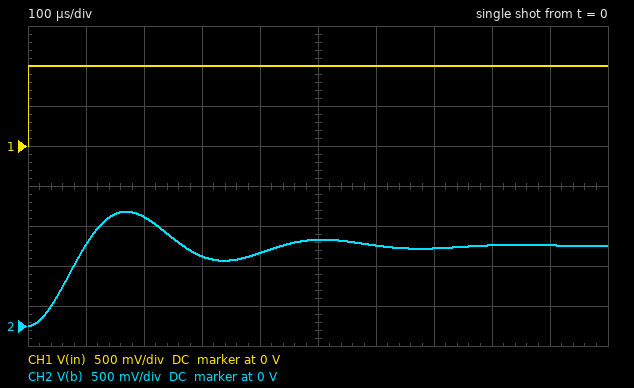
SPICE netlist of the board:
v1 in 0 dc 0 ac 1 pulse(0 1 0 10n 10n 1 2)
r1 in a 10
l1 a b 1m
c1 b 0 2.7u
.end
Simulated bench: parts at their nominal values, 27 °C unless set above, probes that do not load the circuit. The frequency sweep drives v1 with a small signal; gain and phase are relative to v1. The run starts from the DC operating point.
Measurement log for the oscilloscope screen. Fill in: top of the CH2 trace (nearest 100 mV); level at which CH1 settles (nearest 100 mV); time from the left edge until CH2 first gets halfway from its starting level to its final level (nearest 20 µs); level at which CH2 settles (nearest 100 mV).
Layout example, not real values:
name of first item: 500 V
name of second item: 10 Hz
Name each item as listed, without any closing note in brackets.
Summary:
top of the CH2 trace: 1.4 V
level at which CH1 settles: 1.0 V
time from the left edge until CH2 first gets halfway from its starting level to its final level: 60 µs
level at which CH2 settles: 1.0 V
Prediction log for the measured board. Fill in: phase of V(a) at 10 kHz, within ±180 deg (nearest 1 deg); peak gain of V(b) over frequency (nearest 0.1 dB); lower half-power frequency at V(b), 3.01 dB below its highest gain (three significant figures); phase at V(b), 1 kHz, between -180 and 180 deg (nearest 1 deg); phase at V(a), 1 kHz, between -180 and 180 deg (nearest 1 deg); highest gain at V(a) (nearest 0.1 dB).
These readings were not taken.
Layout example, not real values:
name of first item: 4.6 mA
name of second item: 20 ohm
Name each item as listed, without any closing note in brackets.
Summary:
phase of V(a) at 10 kHz, within ±180 deg: 10 deg
peak gain of V(b) over frequency: 6.0 dB
lower half-power frequency at V(b), 3.01 dB below its highest gain: 1.85 kHz
phase at V(b), 1 kHz, between -180 and 180 deg: -11 deg
phase at V(a), 1 kHz, between -180 and 180 deg: -11 deg
highest gain at V(a): 0 dB
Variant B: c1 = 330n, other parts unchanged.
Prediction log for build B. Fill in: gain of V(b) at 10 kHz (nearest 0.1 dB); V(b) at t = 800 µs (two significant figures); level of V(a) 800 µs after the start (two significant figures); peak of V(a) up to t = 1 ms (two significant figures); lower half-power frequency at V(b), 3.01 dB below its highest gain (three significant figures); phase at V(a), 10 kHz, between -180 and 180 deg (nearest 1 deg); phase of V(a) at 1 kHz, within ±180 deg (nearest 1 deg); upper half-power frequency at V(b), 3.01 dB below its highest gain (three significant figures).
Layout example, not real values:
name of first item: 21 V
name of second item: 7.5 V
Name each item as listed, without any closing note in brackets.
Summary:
gain of V(b) at 10 kHz: 8.7 dB
V(b) at t = 800 µs: 980 mV
level of V(a) 800 µs after the start: 1.0 V
peak of V(a) up to t = 1 ms: 1.1 V
lower half-power frequency at V(b), 3.01 dB below its highest gain: 7.85 kHz
phase at V(a), 10 kHz, between -180 and 180 deg: 34 deg
phase of V(a) at 1 kHz, within ±180 deg: -1 deg
upper half-power frequency at V(b), 3.01 dB below its highest gain: 9.45 kHz
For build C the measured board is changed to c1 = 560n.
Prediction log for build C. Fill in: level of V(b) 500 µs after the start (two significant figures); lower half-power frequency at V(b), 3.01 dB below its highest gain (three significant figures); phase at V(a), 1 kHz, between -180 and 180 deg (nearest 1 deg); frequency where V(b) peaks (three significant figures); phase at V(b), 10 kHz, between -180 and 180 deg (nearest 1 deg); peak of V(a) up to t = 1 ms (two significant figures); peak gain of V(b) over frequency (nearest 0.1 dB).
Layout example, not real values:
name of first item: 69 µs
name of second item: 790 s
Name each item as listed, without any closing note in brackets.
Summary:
level of V(b) 500 µs after the start: 1.0 V
lower half-power frequency at V(b), 3.01 dB below its highest gain: 5.77 kHz
phase at V(a), 1 kHz, between -180 and 180 deg: -2 deg
frequency where V(b) peaks: 6.63 kHz
phase at V(b), 10 kHz, between -180 and 180 deg: -164 deg
peak of V(a) up to t = 1 ms: 1.1 V
peak gain of V(b) over frequency: 12.6 dB
